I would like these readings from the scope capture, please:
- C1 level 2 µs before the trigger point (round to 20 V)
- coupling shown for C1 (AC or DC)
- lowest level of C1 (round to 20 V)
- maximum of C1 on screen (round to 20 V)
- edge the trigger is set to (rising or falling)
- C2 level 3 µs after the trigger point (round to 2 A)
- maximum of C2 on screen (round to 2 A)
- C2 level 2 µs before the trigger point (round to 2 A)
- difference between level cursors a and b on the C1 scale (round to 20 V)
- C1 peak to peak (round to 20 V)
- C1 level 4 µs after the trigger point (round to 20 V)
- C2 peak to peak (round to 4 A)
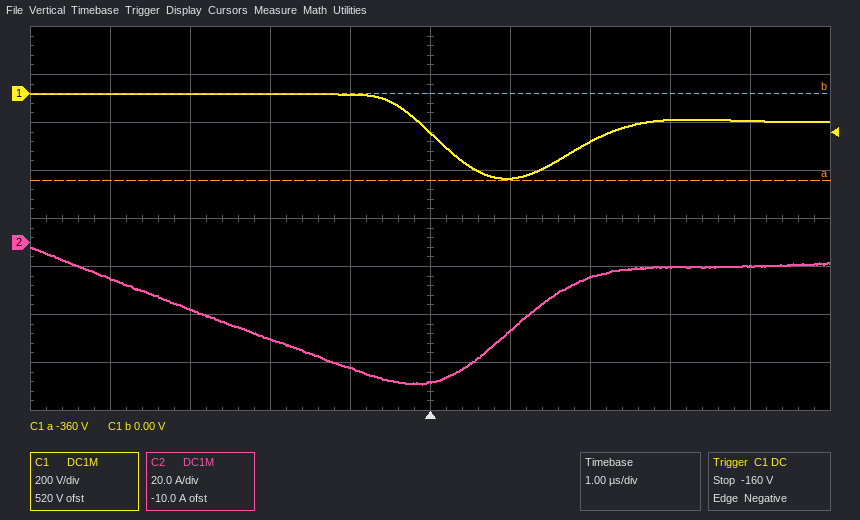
0 V
DC
-360 V
0 V
falling
-10 A
-2 A
-40 A
360 V
360 V
-120 V
56 A
